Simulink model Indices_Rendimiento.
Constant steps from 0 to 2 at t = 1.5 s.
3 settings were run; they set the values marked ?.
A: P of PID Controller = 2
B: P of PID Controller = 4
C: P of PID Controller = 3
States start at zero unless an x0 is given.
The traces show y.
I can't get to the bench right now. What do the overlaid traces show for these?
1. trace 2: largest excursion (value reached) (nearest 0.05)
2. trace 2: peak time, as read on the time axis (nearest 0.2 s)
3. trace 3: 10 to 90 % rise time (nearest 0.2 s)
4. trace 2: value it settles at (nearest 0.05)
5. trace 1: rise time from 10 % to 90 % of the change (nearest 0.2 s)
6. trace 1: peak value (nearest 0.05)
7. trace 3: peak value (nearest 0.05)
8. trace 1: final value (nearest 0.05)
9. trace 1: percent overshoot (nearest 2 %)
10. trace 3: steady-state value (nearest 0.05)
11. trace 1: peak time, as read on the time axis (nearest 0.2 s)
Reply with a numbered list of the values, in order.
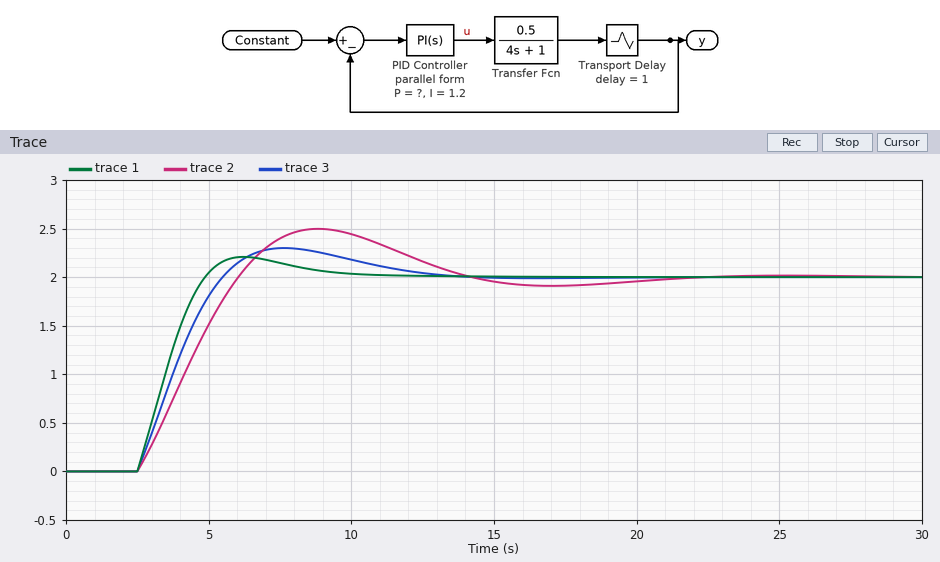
1. 2.50
2. 8.8 s
3. 2.2 s
4. 2.00
5. 1.8 s
6. 2.20
7. 2.30
8. 2.00
9. 10 %
10. 2.00
11. 6.2 s
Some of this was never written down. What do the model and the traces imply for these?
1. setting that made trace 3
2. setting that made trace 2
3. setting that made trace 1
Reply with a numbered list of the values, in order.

1. C
2. A
3. B
